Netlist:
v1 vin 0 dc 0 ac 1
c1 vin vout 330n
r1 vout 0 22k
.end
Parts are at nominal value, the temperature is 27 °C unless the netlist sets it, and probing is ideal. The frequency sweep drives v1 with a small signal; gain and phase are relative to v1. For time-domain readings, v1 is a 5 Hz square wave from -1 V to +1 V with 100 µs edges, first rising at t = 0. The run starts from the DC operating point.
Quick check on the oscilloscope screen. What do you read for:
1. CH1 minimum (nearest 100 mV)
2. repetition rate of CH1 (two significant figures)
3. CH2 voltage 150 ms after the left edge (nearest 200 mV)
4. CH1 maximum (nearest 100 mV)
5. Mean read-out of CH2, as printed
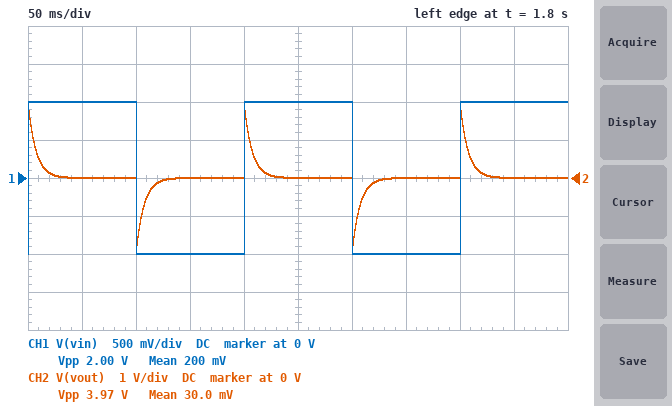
-1.0 V
5.0 Hz
0 V
1.0 V
30.0 mV
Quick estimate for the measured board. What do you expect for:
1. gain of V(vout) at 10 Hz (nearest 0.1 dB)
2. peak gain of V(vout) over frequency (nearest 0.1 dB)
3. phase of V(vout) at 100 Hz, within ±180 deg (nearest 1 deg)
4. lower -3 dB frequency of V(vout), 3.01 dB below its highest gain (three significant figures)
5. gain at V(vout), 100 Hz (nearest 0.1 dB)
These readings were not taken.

-7.6 dB
0 dB
12 deg
21.9 Hz
-0.2 dB
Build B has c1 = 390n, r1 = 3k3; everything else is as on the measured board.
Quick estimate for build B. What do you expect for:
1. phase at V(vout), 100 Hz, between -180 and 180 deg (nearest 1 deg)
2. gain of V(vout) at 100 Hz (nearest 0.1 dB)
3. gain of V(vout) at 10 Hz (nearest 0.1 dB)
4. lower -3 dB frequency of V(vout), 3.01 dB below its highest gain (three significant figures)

51 deg
-4.0 dB
-21.9 dB
124 Hz
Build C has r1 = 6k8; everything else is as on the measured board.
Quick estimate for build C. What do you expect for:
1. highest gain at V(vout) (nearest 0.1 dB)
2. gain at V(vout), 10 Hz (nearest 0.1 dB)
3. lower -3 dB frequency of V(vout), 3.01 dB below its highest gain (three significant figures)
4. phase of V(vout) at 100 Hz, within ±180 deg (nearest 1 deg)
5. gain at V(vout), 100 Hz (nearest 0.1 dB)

0 dB
-17.1 dB
70.9 Hz
35 deg
-1.8 dB
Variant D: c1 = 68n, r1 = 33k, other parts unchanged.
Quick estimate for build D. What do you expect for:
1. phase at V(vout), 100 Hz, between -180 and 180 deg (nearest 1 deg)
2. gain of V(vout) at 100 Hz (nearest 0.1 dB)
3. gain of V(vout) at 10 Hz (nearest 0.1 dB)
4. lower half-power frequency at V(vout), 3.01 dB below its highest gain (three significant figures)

35 deg
-1.8 dB
-17.1 dB
70.9 Hz
